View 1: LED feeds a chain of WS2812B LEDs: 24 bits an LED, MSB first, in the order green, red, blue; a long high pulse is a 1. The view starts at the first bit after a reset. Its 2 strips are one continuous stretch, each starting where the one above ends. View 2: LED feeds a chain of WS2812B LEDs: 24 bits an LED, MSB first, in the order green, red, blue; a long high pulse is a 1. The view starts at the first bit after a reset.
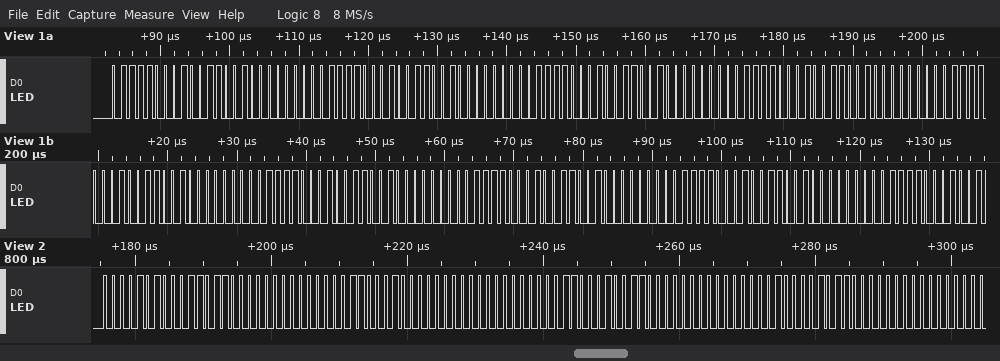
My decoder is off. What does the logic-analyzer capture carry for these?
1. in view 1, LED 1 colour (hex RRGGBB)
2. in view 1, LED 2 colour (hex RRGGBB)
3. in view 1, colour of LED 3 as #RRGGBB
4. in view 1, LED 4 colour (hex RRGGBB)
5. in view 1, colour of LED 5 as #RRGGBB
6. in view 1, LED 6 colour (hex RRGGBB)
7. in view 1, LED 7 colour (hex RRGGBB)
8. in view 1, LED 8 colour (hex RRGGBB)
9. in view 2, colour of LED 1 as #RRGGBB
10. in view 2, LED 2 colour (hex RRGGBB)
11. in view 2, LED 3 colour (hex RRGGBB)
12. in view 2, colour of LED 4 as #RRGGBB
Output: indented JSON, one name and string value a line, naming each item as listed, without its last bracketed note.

{
  "in view 1, LED 1 colour": "#997800",
  "in view 1, LED 2 colour": "#997800",
  "in view 1, colour of LED 3 as #RRGGBB": "#997800",
  "in view 1, LED 4 colour": "#997800",
  "in view 1, colour of LED 5 as #RRGGBB": "#997800",
  "in view 1, LED 6 colour": "#997800",
  "in view 1, LED 7 colour": "#997800",
  "in view 1, LED 8 colour": "#997800",
  "in view 2, colour of LED 1 as #RRGGBB": "#360A00",
  "in view 2, LED 2 colour": "#200600",
  "in view 2, LED 3 colour": "#130300",
  "in view 2, colour of LED 4 as #RRGGBB": "#0B0100"
}
